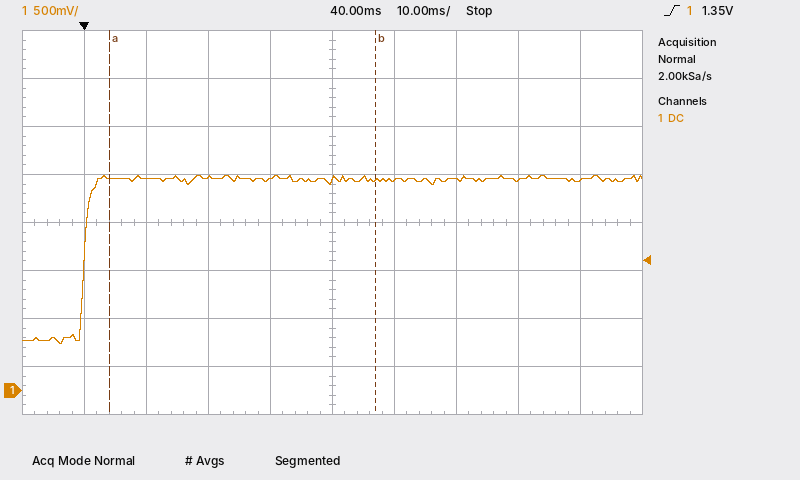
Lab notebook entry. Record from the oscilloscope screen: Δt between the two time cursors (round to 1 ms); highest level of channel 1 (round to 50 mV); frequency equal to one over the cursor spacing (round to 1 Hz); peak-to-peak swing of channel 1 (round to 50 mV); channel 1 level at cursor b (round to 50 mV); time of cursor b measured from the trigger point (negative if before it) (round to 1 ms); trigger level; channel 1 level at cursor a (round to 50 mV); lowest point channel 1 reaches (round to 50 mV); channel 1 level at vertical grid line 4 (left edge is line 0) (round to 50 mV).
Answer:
43 ms
2.25 V
23 Hz
1.75 V
2.20 V
+47 ms
1.35 V
2.20 V
500 mV
2.20 V
